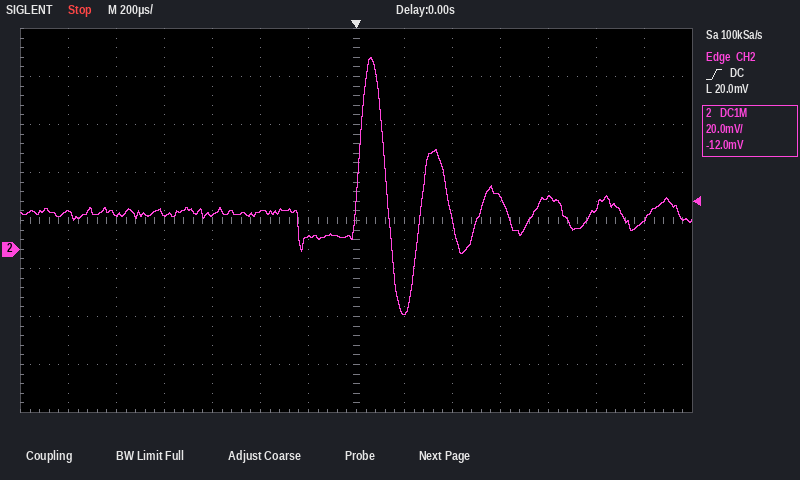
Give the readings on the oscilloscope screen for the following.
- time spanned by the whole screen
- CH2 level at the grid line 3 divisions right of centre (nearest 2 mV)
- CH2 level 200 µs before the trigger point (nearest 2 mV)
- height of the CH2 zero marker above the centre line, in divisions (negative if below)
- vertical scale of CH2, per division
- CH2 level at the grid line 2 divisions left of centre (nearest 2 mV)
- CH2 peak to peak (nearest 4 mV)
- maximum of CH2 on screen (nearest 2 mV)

2.8 ms
22 mV
6 mV
-0.6 div
20 mV
16 mV
108 mV
80 mV
